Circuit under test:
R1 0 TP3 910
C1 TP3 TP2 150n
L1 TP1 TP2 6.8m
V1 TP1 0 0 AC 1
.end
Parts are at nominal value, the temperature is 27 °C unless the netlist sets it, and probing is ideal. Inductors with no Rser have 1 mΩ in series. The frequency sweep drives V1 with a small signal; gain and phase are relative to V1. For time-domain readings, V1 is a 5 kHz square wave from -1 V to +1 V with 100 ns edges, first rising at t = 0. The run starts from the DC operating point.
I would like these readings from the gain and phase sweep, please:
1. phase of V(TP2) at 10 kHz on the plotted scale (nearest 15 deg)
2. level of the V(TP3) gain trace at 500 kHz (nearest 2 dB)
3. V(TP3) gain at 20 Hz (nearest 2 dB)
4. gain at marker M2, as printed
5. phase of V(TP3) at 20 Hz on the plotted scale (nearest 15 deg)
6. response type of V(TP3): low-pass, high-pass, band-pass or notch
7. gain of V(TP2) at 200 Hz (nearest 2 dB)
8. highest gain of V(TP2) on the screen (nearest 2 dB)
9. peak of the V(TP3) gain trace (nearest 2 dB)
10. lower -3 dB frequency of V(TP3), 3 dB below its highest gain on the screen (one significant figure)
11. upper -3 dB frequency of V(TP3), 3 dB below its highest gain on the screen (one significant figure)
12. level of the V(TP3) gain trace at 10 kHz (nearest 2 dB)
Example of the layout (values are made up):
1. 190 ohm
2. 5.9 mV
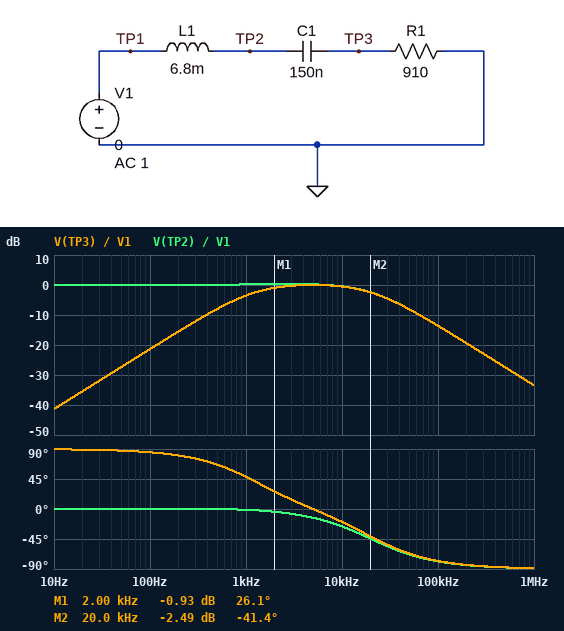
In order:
1. -30 deg
2. -28 dB
3. -36 dB
4. -2.49 dB
5. 90 deg
6. band-pass
7. 0 dB
8. 0 dB
9. 0 dB
10. 1 kHz
11. 20 kHz
12. 0 dB
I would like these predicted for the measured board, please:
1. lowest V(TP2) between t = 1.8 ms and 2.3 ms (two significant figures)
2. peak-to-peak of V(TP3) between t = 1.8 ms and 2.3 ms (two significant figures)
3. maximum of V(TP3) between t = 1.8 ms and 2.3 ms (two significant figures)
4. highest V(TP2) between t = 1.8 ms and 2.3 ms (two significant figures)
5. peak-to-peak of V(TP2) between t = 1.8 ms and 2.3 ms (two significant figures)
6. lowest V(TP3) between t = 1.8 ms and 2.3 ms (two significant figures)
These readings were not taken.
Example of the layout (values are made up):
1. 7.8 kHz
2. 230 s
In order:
1. -1.1 V
2. 2.4 V
3. 1.2 V
4. 1.1 V
5. 2.1 V
6. -1.2 V
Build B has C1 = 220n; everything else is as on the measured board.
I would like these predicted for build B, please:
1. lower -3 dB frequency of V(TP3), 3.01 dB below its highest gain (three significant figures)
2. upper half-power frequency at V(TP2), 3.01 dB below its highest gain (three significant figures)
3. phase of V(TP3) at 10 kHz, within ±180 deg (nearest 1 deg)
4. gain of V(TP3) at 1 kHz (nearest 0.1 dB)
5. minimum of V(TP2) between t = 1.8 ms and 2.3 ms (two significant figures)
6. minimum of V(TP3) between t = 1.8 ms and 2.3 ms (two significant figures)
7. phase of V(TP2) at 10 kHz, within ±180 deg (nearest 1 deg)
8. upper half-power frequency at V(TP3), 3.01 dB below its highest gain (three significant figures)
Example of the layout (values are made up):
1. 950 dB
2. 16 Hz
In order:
1. 767 Hz
2. 20.9 kHz
3. -21 deg
4. -1.9 dB
5. -1.0 V
6. -1.1 V
7. -26 deg
8. 22.1 kHz
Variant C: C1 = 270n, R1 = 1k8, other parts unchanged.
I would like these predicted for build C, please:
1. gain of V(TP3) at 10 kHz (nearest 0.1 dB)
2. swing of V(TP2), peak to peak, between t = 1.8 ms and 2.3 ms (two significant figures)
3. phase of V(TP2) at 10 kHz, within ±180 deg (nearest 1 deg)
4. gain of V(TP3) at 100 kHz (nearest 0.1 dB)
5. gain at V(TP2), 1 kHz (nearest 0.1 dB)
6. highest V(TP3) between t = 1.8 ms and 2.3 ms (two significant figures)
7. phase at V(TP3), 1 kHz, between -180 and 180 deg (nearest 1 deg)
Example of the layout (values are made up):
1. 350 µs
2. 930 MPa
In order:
1. -0.2 dB
2. 2.0 V
3. -13 deg
4. -8.2 dB
5. 0.1 dB
6. 1.1 V
7. 17 deg
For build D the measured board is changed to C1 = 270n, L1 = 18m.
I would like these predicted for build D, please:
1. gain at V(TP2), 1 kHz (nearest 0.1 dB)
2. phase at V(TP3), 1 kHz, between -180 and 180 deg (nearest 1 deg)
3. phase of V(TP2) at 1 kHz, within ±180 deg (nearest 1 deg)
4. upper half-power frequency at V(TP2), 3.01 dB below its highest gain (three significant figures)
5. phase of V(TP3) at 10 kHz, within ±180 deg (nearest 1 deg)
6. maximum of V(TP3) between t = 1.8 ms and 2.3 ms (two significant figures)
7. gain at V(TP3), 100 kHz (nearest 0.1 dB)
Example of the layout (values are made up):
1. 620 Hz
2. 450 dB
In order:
1. 0.5 dB
2. 28 deg
3. -5 deg
4. 7.84 kHz
5. -50 deg
6. 990 mV
7. -21.9 dB
